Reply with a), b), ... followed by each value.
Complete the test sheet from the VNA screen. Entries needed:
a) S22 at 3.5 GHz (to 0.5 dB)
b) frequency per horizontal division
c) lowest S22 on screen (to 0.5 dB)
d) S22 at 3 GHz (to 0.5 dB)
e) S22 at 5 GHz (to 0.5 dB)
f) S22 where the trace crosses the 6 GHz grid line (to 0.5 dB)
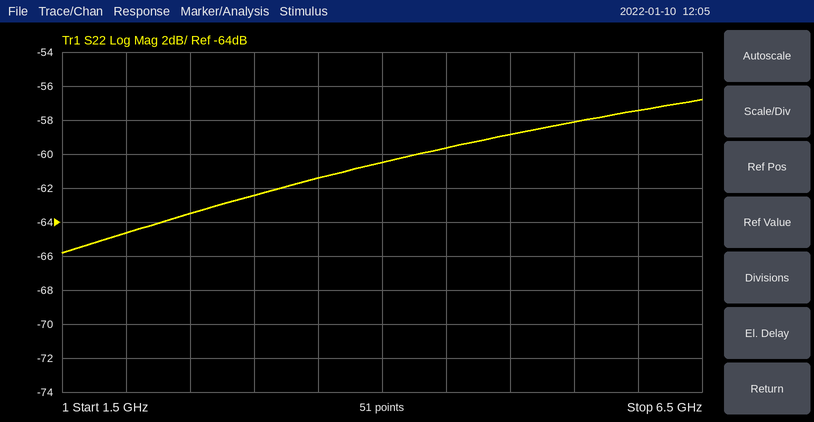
a) -61.5 dB
b) 500 MHz
c) -66.0 dB
d) -62.5 dB
e) -59.0 dB
f) -57.5 dB
